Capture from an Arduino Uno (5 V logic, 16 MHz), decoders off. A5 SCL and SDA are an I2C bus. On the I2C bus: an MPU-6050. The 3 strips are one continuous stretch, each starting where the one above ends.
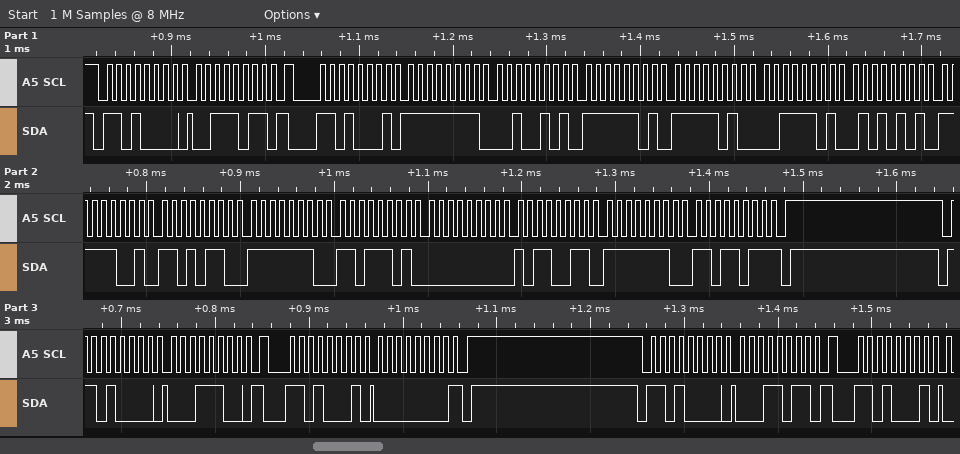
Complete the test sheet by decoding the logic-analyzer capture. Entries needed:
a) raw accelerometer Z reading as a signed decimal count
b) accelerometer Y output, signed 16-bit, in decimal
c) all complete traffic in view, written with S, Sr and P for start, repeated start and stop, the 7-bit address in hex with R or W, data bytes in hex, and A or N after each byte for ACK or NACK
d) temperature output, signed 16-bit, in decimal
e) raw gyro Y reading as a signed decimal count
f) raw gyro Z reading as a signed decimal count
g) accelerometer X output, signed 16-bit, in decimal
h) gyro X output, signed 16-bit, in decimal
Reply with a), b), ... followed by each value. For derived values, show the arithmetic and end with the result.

a) 0x3D55 = 15701
b) 0xFDFA = -518
c) S 68W A 3B A Sr 68R A FF A 25 A FD A FA A 3D A 55 A F9 A D6 A FE A DD A 00 A B3 A FE A DB N P S 68W A 1C A Sr 68R A 00 N P S 68W A 1B A Sr 68R A
d) 0xF9D6 = -1578
e) 0x00B3 = 179
f) 0xFEDB = -293
g) 0xFF25 = -219
h) 0xFEDD = -291
